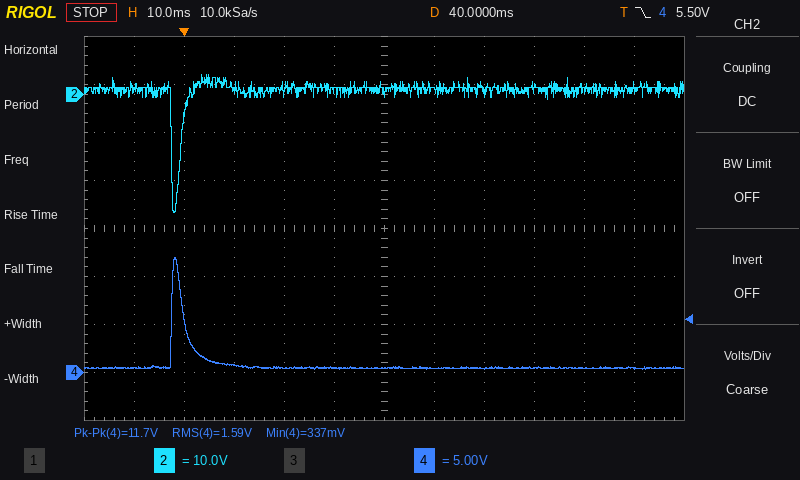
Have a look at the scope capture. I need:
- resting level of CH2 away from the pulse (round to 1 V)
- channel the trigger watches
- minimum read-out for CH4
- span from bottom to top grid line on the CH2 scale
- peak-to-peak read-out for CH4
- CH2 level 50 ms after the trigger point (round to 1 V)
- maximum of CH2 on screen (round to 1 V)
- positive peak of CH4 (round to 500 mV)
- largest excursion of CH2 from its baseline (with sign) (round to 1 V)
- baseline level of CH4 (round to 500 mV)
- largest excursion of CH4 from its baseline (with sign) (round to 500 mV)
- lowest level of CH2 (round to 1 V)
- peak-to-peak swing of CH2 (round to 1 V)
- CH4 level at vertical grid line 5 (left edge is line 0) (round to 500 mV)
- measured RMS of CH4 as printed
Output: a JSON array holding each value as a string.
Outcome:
["1 V", "CH4", "337 mV", "80 V", "11.7 V", "1 V", "4 V", "12.0 V", "-26 V", "500 mV", "+11.5 V", "-25 V", "29 V", "500 mV", "1.59 V"]
